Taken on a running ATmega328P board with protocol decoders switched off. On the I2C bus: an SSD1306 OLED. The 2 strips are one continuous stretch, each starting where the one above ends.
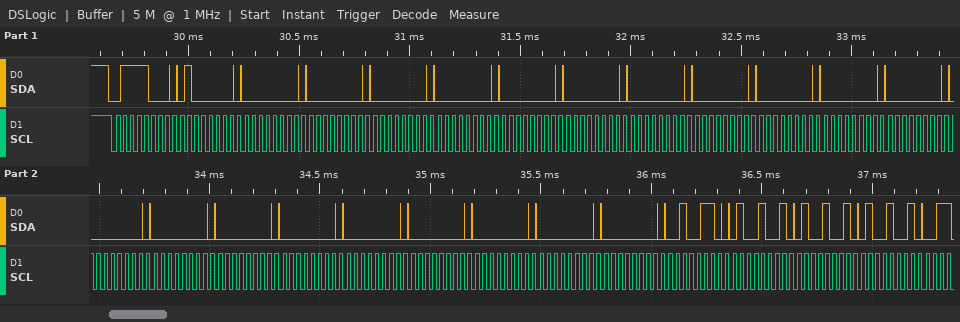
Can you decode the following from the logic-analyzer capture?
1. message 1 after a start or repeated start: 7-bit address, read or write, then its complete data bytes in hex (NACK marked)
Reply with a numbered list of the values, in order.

1. 0x3C write: 40 00 00 00 00 00 00 00 00 00 00 00 00 00 00 00 00 00 00 00 00 26 49 49 49
